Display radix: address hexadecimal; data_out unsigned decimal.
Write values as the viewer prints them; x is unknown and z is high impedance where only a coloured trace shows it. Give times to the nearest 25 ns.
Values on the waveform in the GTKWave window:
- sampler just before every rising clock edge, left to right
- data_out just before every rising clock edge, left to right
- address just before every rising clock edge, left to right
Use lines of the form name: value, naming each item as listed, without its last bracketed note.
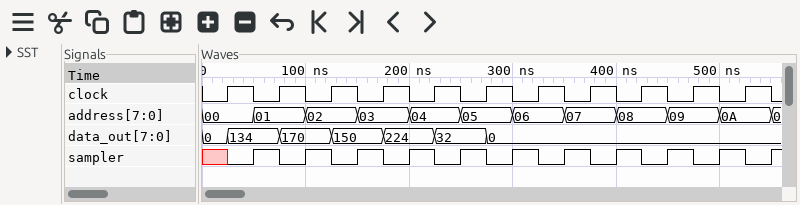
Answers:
sampler just before every rising clock edge, left to right: x 1 1 1 1 1 1 1 1 1 1
data_out just before every rising clock edge, left to right: 0, 134, 170, 150, 224, 32, 0, 0, 0, 0, 0
address just before every rising clock edge, left to right: 00, 01, 02, 03, 04, 05, 06, 07, 08, 09, 0A
